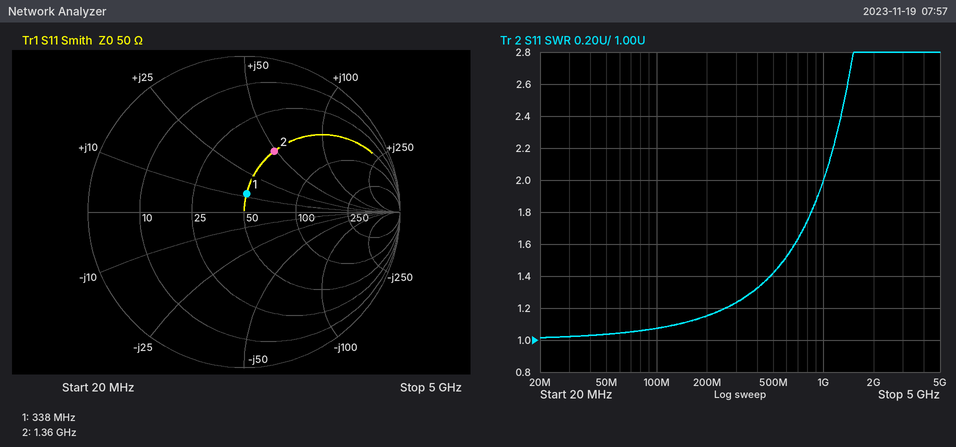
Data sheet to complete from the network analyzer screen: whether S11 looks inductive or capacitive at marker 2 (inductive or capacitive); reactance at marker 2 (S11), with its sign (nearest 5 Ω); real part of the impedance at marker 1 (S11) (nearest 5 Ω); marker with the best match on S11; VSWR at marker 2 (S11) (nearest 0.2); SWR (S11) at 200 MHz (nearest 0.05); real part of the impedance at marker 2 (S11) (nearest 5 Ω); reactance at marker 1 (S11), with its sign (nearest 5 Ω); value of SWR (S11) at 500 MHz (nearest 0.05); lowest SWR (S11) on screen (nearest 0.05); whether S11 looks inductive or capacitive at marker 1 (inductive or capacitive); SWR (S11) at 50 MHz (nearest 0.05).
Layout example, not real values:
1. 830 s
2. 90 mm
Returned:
1. inductive
2. +50 Ω
3. 50 Ω
4. marker 1
5. 2.6
6. 1.15
7. 50 Ω
8. +10 Ω
9. 1.40
10. 1.00
11. inductive
12. 1.05
